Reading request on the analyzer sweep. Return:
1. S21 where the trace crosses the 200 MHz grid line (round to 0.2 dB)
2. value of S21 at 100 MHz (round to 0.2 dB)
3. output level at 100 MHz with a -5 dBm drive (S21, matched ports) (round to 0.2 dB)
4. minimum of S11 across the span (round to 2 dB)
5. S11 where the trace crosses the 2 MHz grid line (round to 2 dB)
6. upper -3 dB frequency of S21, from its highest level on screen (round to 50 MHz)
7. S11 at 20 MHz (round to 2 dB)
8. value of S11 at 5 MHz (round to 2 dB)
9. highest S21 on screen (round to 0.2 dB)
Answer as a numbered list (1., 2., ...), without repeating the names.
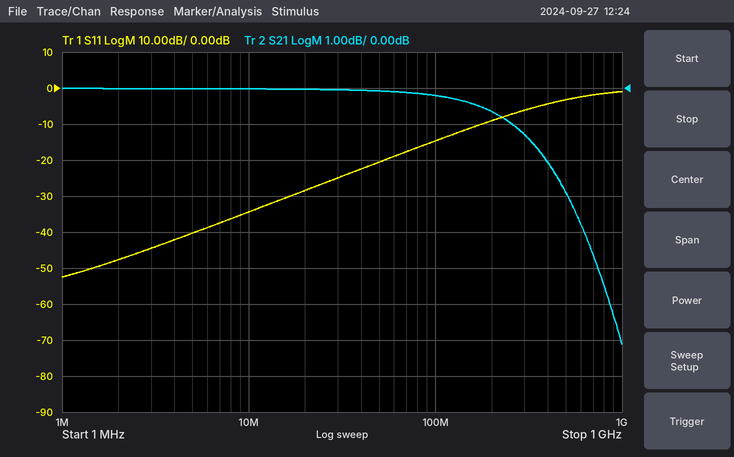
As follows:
1. -0.6 dB
2. -0.2 dB
3. -5.2 dBm
4. -52 dB
5. -48 dB
6. 500 MHz
7. -28 dB
8. -40 dB
9. 0.0 dB
